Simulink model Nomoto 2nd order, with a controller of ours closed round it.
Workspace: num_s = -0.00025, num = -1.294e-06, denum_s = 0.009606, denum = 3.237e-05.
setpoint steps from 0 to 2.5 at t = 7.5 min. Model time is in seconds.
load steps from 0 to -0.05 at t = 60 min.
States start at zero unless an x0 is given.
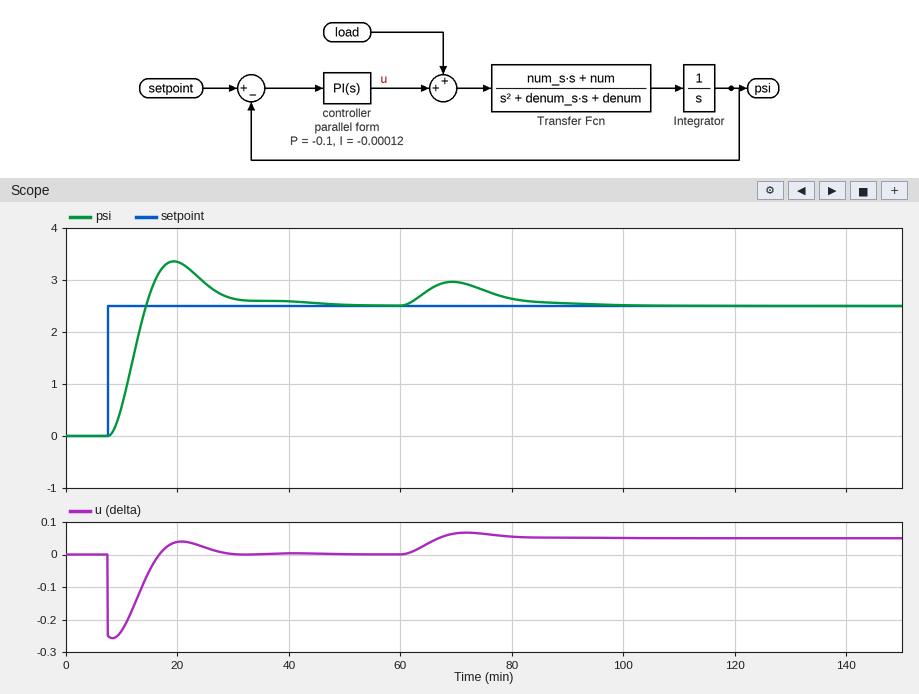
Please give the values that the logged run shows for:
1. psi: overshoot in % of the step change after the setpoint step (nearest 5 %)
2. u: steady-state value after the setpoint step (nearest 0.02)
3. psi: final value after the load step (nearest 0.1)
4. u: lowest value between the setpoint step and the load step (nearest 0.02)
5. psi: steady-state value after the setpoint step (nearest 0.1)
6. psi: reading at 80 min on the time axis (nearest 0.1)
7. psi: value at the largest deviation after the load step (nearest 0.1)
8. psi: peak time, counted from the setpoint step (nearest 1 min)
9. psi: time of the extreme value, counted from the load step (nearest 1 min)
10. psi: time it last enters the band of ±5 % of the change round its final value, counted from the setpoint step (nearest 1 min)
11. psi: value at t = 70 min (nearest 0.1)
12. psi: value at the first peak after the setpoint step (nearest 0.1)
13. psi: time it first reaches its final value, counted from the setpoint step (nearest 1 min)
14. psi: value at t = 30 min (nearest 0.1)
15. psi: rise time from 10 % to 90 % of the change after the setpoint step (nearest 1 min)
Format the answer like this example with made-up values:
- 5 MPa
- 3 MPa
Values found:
- 35 %
- 0.00
- 2.5
- -0.26
- 2.5
- 2.6
- 3.0
- 12 min
- 9 min
- 23 min
- 3.0
- 3.4
- 7 min
- 2.6
- 5 min
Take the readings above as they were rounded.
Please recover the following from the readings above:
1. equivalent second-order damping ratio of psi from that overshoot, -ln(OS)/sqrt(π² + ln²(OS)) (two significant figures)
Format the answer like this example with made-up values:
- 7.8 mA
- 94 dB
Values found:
- 0.32
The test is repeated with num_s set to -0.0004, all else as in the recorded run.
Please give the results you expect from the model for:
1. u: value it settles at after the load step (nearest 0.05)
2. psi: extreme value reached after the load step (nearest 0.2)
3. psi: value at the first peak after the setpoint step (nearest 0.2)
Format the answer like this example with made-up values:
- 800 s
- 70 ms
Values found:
- 0.05
- 3.0
- 3.0
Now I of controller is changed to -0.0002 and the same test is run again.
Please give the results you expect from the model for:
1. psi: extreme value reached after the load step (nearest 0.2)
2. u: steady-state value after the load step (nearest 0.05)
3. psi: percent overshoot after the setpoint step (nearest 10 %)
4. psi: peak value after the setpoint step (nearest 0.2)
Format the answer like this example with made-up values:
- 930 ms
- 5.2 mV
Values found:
- 3.0
- 0.05
- 50 %
- 3.8
